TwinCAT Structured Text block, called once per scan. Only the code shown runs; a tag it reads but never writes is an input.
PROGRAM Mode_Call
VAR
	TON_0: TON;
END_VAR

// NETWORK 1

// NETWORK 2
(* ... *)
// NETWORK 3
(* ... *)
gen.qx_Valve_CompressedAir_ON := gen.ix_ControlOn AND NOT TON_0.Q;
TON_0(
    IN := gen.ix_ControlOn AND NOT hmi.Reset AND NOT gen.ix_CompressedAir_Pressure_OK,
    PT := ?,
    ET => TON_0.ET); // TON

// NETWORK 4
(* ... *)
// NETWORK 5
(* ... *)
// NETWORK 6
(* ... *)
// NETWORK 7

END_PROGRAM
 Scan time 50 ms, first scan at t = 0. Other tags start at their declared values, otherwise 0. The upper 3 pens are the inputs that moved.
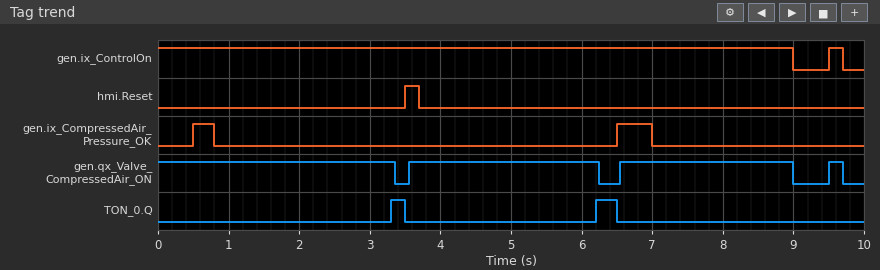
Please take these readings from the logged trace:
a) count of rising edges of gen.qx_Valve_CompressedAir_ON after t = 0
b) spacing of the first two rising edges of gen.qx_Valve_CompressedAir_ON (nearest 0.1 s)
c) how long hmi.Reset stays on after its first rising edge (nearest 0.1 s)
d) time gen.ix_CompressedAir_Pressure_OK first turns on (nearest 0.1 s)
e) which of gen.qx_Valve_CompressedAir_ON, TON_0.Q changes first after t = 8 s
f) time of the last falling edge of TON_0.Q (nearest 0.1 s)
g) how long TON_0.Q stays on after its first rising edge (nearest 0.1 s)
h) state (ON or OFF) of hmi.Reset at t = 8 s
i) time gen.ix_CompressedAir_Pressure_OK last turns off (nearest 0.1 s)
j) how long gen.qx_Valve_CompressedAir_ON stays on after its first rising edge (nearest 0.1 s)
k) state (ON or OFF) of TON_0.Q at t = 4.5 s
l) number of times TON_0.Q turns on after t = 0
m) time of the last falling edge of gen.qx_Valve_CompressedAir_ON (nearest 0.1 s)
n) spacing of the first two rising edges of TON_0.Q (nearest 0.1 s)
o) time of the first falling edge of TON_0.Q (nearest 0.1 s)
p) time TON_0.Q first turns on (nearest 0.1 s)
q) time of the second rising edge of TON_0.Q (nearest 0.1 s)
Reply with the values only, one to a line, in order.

3
3.0 s
0.2 s
0.5 s
gen.qx_Valve_CompressedAir_ON
6.5 s
0.2 s
OFF
7.0 s
2.7 s
OFF
2
9.7 s
2.9 s
3.5 s
3.3 s
6.2 s
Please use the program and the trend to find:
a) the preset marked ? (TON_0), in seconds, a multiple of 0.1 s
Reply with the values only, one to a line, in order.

2.5 s
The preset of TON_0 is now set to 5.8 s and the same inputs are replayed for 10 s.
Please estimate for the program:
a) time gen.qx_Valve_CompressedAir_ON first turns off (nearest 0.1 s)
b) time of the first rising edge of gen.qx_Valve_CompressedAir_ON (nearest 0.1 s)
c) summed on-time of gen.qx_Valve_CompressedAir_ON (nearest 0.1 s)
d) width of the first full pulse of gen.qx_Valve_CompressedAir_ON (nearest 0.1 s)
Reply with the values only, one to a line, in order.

9.0 s
9.5 s
9.2 s
0.2 s
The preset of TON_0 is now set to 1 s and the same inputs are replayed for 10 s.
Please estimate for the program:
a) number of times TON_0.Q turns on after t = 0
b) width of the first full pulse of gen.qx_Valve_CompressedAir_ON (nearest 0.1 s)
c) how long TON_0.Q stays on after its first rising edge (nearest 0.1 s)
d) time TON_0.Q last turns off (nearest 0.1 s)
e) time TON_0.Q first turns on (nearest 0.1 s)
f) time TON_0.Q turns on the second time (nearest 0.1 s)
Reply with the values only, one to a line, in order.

3
1.2 s
1.7 s
9.0 s
1.8 s
4.7 s
